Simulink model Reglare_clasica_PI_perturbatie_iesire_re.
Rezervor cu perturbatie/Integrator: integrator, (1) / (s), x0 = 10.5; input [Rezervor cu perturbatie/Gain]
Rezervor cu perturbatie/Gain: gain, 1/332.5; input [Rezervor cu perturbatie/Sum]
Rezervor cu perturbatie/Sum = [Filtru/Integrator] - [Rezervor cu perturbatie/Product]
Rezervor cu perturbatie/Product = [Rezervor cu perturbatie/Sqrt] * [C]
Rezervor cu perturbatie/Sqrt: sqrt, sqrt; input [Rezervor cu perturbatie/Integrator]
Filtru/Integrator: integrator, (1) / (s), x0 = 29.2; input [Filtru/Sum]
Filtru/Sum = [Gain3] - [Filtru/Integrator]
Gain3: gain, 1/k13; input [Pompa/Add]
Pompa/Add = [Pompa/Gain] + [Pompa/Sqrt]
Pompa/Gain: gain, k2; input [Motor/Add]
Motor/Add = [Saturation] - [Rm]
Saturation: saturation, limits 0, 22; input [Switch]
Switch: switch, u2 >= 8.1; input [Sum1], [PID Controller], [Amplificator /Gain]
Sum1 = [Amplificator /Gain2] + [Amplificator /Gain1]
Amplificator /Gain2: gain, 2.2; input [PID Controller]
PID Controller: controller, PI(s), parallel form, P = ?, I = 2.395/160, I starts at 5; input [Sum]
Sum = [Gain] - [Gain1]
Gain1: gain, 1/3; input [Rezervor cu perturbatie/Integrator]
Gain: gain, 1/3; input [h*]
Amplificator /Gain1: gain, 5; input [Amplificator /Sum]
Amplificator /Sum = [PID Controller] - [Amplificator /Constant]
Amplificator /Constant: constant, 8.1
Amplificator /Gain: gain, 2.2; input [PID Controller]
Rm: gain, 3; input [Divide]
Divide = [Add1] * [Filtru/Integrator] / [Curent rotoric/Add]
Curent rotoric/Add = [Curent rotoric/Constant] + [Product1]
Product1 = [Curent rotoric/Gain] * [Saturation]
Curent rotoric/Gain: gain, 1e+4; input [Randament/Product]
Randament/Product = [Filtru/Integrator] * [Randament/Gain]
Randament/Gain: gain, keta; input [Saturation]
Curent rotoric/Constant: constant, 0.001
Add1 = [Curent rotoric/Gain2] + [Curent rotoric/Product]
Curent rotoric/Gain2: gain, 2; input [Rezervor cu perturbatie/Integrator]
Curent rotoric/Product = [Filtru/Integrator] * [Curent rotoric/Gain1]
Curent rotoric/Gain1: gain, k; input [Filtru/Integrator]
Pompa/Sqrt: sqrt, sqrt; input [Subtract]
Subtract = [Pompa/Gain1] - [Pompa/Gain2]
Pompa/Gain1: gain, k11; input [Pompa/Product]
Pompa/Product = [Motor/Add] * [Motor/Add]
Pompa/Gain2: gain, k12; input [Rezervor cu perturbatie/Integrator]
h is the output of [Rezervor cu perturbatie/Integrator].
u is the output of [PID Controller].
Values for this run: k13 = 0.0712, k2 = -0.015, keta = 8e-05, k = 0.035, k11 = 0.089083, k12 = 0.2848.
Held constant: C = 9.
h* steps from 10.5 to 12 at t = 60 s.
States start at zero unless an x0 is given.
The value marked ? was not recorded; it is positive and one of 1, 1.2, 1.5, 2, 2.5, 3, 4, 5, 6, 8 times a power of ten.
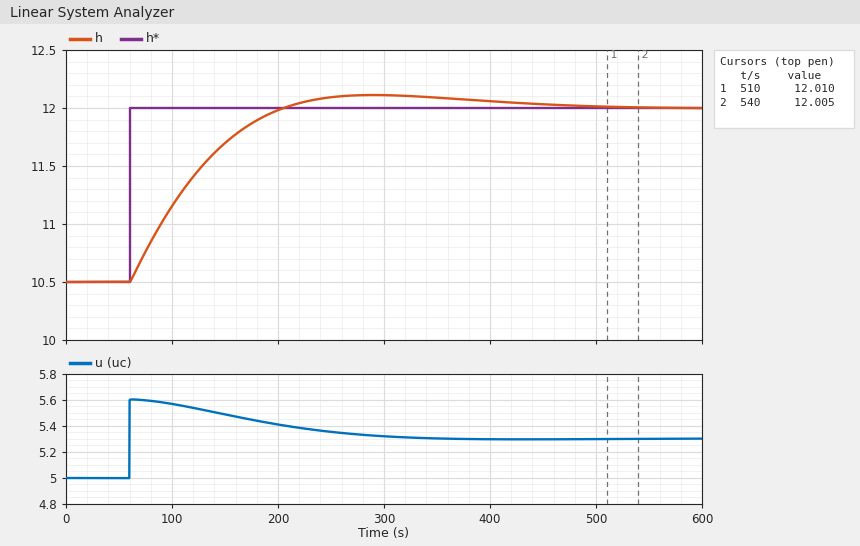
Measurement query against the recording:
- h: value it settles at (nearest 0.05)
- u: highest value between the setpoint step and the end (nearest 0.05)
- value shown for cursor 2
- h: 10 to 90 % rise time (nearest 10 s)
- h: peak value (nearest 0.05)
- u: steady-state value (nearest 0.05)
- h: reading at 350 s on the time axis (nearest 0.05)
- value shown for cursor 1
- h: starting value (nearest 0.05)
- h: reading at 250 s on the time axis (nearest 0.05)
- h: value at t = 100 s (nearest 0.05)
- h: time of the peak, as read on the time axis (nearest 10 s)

12.00
5.60
12.005
100 s
12.10
5.30
12.10
12.010
10.50
12.10
11.15
290 s
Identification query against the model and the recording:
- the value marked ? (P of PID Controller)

1.2
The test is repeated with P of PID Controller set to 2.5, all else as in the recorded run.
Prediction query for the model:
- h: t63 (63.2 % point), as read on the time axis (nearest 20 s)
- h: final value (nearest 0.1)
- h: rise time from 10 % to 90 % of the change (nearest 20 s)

100 s
12.0
80 s
